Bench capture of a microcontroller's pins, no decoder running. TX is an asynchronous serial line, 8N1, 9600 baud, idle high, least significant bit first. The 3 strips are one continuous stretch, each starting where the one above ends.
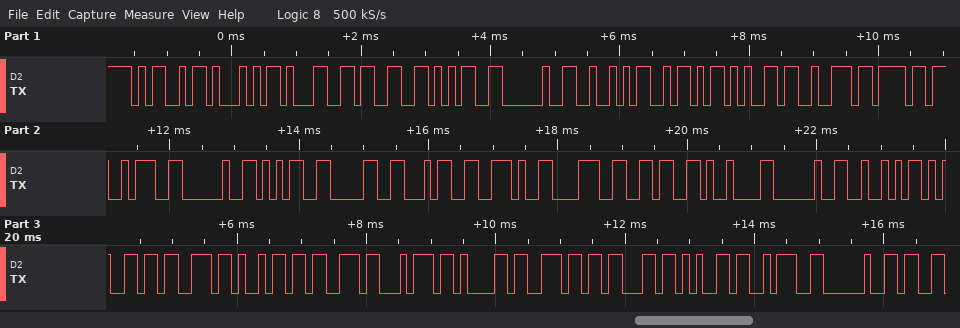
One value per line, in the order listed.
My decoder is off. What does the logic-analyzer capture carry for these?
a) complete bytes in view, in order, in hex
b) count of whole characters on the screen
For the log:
4D 51 31 33 35 20 52 5A 65 72 6F 3A 20 35 30 34 2E 38 36 09 20 52 65 73 69 73 74 61 6E 63 65 3A 20
33
